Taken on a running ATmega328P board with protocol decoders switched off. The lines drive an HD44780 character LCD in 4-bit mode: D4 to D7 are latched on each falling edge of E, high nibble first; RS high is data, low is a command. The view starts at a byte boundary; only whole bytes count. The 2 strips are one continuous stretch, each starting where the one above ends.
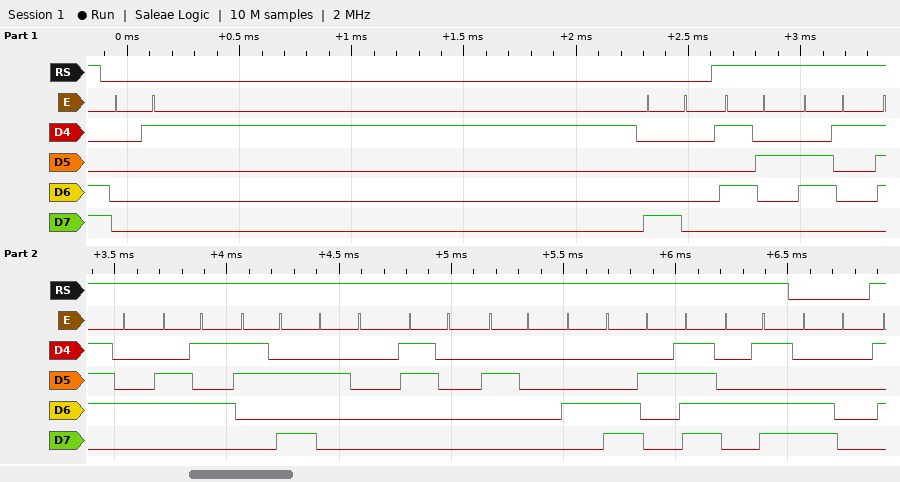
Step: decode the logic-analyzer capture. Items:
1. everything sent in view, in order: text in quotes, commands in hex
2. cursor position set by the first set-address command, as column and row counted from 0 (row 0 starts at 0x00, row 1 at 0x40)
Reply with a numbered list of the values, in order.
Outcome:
1. 0x01 0x80 "Rate: 0 L/M" 0xC0
2. column 0, row 0
